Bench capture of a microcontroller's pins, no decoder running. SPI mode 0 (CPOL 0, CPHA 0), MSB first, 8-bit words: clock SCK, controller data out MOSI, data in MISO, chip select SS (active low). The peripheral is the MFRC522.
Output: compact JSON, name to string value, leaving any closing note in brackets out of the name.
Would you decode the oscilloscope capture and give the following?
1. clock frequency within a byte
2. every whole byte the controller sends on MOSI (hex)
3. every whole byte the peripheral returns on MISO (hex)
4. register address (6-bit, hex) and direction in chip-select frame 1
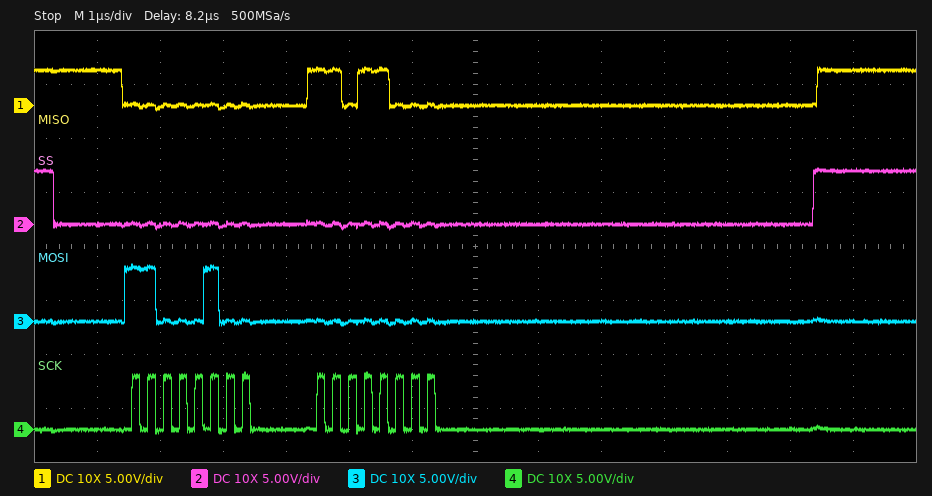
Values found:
{"clock frequency within a byte": "4 MHz", "every whole byte the controller sends on MOSI": "C4 00", "every whole byte the peripheral returns on MISO": "00 D8", "register address (6-bit, hex) and direction in chip-select frame 1": "0x22 read"}
